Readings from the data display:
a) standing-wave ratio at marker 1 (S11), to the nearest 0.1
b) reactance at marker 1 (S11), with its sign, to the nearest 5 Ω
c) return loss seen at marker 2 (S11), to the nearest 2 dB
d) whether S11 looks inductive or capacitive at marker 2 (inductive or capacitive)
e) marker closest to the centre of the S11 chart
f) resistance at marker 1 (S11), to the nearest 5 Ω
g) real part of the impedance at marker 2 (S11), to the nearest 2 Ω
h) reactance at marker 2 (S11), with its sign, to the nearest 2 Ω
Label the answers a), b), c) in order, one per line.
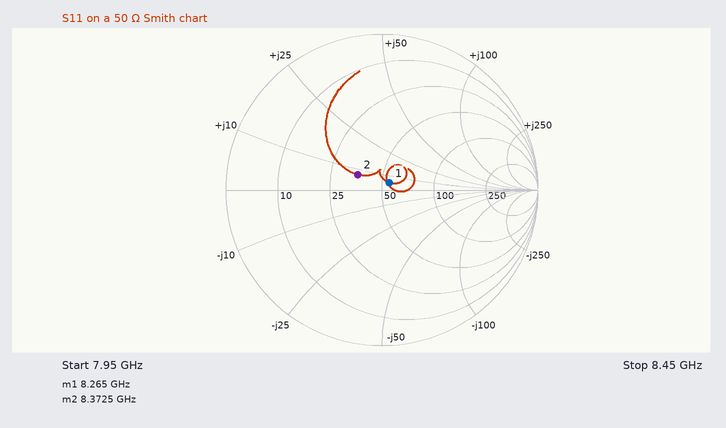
a) 1.1
b) +5 Ω
c) 14 dB
d) inductive
e) marker 1
f) 55 Ω
g) 36 Ω
h) +8 Ω
